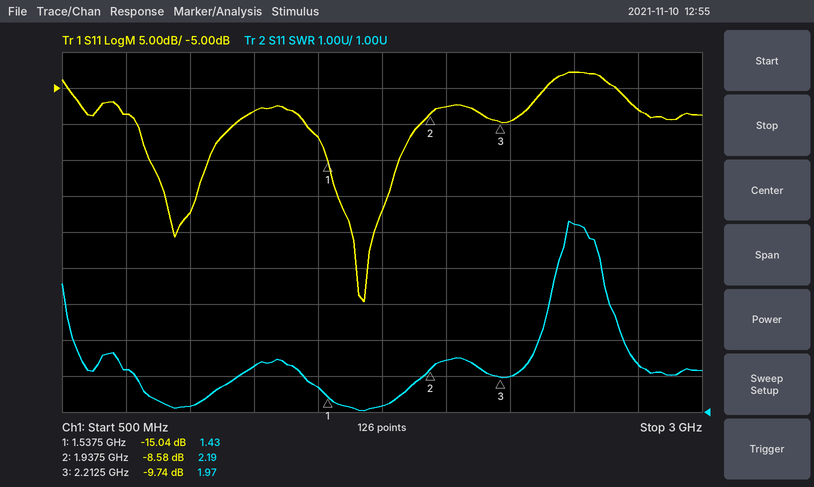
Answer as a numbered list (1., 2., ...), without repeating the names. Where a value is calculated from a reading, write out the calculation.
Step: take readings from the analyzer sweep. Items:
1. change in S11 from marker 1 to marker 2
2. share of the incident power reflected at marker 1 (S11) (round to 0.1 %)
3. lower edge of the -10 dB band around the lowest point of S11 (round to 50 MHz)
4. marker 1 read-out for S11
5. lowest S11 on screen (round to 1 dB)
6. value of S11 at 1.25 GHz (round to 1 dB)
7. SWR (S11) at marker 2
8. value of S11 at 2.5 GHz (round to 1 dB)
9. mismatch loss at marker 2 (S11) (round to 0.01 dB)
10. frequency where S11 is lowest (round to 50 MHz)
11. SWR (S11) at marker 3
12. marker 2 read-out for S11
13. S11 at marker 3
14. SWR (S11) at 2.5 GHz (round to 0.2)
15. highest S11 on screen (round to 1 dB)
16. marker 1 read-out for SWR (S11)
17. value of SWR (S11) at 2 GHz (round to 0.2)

1. -8.58 − (-15.04) = 6.46 dB
2. 10^(-15.04/10) ≈ 3.1 %
3. 1.45 GHz
4. -15.04 dB
5. -35 dB
6. -8 dB
7. 2.19
8. -3 dB
9. −10 log10(1 − 10^(-8.58/10)) ≈ 0.65 dB
10. 1.70 GHz
11. 1.97
12. -8.58 dB
13. -9.74 dB
14. 6.2
15. -3 dB
16. 1.43
17. 2.4
